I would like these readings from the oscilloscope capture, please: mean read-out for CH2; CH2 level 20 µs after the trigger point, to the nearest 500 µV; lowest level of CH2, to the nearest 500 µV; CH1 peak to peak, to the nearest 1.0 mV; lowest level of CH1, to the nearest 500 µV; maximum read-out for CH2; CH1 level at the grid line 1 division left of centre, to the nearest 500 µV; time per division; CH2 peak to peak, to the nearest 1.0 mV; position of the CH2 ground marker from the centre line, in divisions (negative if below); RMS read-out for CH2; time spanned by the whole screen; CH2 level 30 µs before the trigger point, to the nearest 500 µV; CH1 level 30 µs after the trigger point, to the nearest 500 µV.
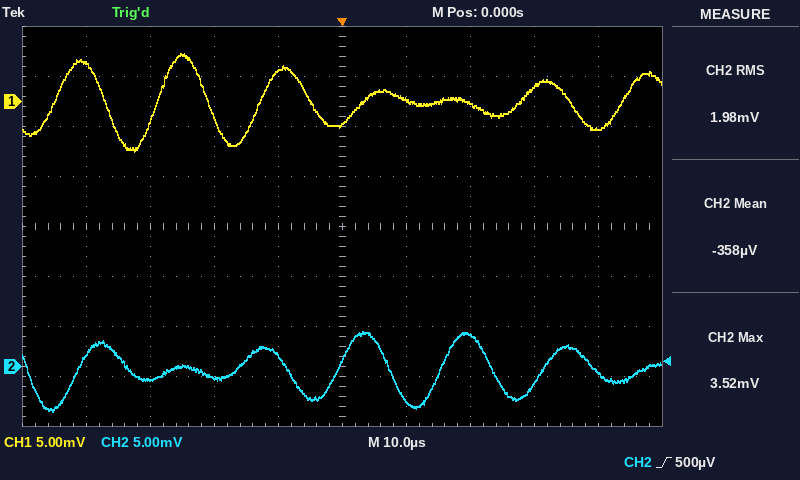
-358 µV
3.0 mV
-4.5 mV
10.0 mV
-5.0 mV
3.52 mV
3.0 mV
10 µs
8.0 mV
-2.8 div
1.98 mV
100 µs
-1.5 mV
1.5 mV
